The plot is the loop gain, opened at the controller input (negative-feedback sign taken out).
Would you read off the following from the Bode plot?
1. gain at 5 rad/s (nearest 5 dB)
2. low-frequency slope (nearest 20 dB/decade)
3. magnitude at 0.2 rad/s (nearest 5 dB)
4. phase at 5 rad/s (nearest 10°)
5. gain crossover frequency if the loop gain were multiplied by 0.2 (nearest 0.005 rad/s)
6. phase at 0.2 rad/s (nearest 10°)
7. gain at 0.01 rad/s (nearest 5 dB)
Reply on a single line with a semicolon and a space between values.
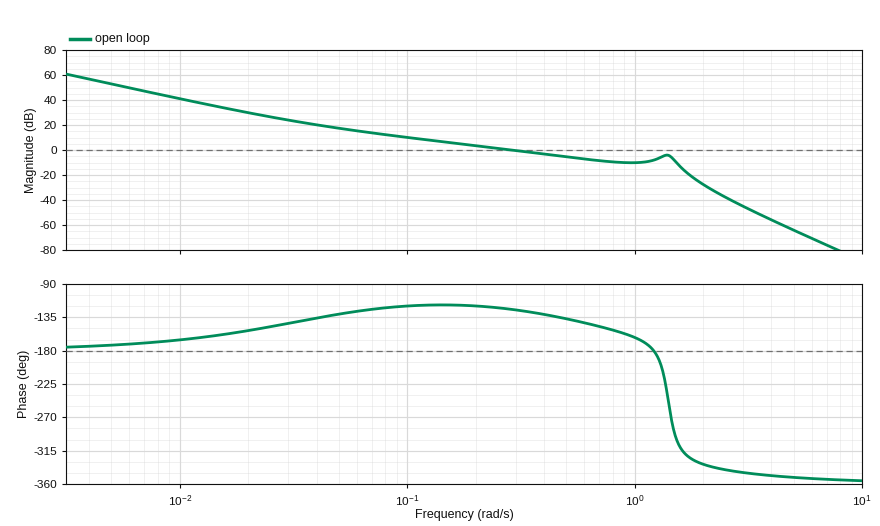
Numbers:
-65 dB; -40 dB/decade; 5 dB; -350°; 0.070 rad/s; -120°; 40 dB
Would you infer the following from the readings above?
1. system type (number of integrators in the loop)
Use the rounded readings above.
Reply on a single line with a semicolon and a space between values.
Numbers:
2
